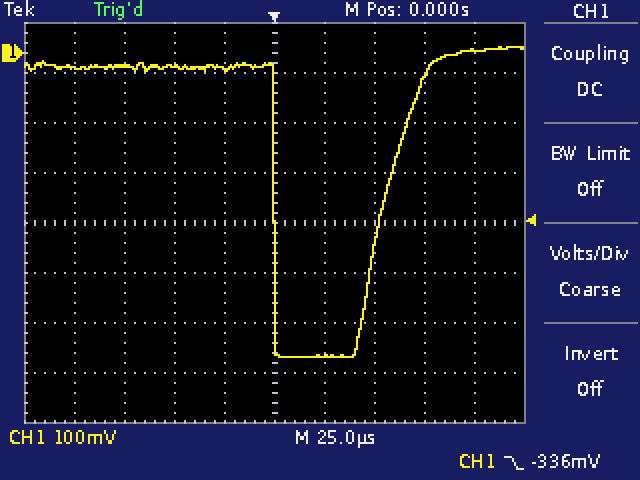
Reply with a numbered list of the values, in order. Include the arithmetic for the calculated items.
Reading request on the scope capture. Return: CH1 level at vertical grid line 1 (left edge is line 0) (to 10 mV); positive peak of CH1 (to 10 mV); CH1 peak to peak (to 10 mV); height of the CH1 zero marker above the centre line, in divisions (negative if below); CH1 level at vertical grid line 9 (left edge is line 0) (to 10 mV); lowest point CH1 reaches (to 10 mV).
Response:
1. -30 mV
2. 10 mV
3. 10 mV − (-610 mV) = 620 mV
4. +3.4 div
5. 10 mV
6. -610 mV
